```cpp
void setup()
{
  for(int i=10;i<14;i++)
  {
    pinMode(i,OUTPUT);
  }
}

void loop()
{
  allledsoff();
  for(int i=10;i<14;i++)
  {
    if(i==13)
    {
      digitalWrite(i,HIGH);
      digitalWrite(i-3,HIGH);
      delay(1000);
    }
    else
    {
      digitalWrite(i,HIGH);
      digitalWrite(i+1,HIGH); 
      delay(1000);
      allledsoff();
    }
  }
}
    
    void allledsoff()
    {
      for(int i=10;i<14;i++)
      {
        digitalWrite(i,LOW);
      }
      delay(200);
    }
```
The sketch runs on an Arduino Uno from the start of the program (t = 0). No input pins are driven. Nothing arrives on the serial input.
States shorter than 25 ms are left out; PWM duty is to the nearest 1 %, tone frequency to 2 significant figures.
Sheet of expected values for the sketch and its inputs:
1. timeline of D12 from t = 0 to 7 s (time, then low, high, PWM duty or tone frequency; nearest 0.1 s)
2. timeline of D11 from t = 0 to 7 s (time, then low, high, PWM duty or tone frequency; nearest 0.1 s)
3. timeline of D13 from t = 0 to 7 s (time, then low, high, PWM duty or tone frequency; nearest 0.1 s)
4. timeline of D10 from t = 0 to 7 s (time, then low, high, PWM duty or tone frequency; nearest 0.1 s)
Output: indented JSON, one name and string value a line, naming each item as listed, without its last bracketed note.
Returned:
{
  "timeline of D12 from t = 0 to 7 s": "0 s low; 1.4 s high; 2.4 s low; 2.6 s high; 3.6 s low; 6.2 s high",
  "timeline of D11 from t = 0 to 7 s": "0 s low; 0.2 s high; 1.2 s low; 1.4 s high; 2.4 s low; 5 s high; 6 s low; 6.2 s high",
  "timeline of D13 from t = 0 to 7 s": "0 s low; 2.6 s high; 3.6 s low; 3.8 s high; 4.8 s low",
  "timeline of D10 from t = 0 to 7 s": "0 s low; 0.2 s high; 1.2 s low; 3.8 s high; 4.8 s low; 5 s high; 6 s low"
}
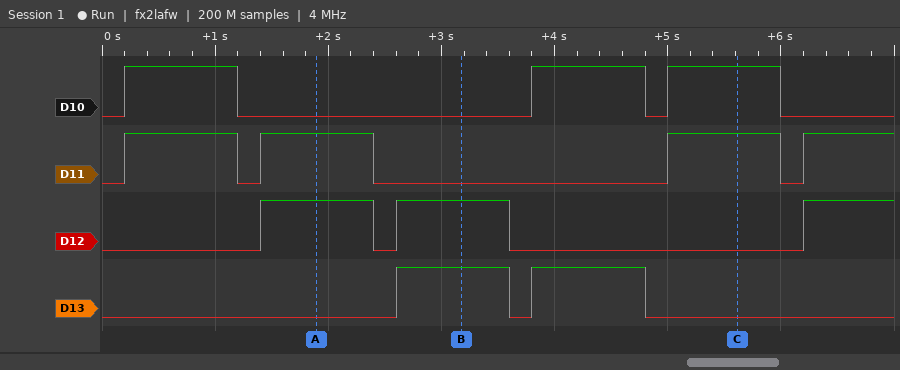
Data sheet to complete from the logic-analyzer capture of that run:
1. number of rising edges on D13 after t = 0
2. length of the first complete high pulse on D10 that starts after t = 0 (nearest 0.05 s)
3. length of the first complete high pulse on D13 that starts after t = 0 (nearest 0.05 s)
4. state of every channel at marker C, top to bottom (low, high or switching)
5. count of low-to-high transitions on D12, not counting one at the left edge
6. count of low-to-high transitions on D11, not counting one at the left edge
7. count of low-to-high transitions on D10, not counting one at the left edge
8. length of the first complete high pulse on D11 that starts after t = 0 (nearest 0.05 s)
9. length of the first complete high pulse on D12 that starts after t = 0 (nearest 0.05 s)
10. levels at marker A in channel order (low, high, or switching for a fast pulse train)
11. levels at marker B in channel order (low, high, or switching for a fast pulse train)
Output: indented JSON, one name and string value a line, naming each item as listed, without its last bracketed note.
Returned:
{
  "number of rising edges on D13 after t = 0": "2",
  "length of the first complete high pulse on D10 that starts after t = 0": "1.00 s",
  "length of the first complete high pulse on D13 that starts after t = 0": "1.00 s",
  "state of every channel at marker C, top to bottom": "D10 high, D11 high, D12 low, D13 low",
  "count of low-to-high transitions on D12, not counting one at the left edge": "3",
  "count of low-to-high transitions on D11, not counting one at the left edge": "4",
  "count of low-to-high transitions on D10, not counting one at the left edge": "3",
  "length of the first complete high pulse on D11 that starts after t = 0": "1.00 s",
  "length of the first complete high pulse on D12 that starts after t = 0": "1.00 s",
  "levels at marker A in channel order": "D10 low, D11 high, D12 high, D13 low",
  "levels at marker B in channel order": "D10 low, D11 low, D12 high, D13 high"
}
